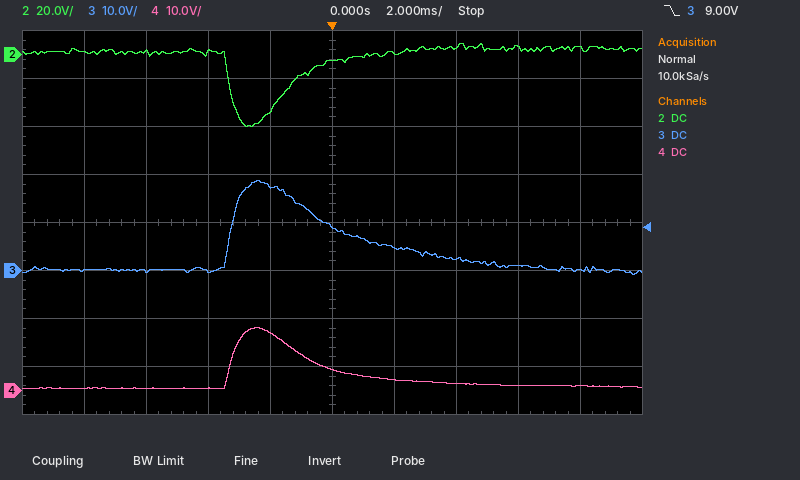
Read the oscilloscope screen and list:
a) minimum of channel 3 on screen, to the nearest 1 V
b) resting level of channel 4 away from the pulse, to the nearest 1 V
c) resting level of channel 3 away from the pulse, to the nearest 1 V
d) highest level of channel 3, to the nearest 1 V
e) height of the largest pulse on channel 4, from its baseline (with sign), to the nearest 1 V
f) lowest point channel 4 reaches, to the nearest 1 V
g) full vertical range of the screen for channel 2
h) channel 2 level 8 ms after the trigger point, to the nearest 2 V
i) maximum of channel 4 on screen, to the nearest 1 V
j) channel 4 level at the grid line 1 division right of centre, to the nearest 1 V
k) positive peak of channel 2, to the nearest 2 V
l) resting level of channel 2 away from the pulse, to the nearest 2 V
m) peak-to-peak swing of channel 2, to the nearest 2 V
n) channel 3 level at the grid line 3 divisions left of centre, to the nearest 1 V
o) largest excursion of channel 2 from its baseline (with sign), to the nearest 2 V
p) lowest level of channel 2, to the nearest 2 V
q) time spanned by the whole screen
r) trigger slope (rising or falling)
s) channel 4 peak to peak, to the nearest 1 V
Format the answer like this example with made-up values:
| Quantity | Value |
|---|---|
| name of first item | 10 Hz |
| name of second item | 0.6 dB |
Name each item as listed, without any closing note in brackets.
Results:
| Quantity | Value |
|---|---|
| minimum of channel 3 on screen, to the nearest 1 V | -1 V |
| resting level of channel 4 away from the pulse, to the nearest 1 V | 1 V |
| resting level of channel 3 away from the pulse, to the nearest 1 V | 0 V |
| highest level of channel 3, to the nearest 1 V | 19 V |
| height of the largest pulse on channel 4, from its baseline (with sign), to the nearest 1 V | +12 V |
| lowest point channel 4 reaches, to the nearest 1 V | 0 V |
| full vertical range of the screen for channel 2 | 160 V |
| channel 2 level 8 ms after the trigger point, to the nearest 2 V | 2 V |
| maximum of channel 4 on screen, to the nearest 1 V | 13 V |
| channel 4 level at the grid line 1 division right of centre, to the nearest 1 V | 2 V |
| positive peak of channel 2, to the nearest 2 V | 4 V |
| resting level of channel 2 away from the pulse, to the nearest 2 V | 2 V |
| peak-to-peak swing of channel 2, to the nearest 2 V | 34 V |
| channel 3 level at the grid line 3 divisions left of centre, to the nearest 1 V | 0 V |
| largest excursion of channel 2 from its baseline (with sign), to the nearest 2 V | -32 V |
| lowest level of channel 2, to the nearest 2 V | -30 V |
| time spanned by the whole screen | 20 ms |
| trigger slope | falling |
| channel 4 peak to peak, to the nearest 1 V | 13 V |
